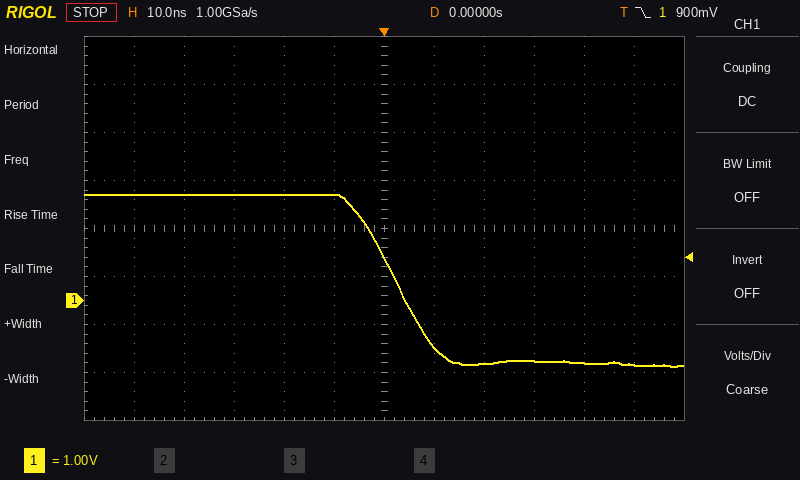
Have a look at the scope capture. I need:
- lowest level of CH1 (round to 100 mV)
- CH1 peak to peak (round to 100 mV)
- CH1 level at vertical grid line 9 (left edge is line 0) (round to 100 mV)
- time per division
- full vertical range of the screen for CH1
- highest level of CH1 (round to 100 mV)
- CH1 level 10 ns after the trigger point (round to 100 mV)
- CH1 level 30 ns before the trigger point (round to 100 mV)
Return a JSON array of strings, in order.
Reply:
["-1.4 V", "3.6 V", "-1.3 V", "10 ns", "8 V", "2.2 V", "-1.0 V", "2.2 V"]
